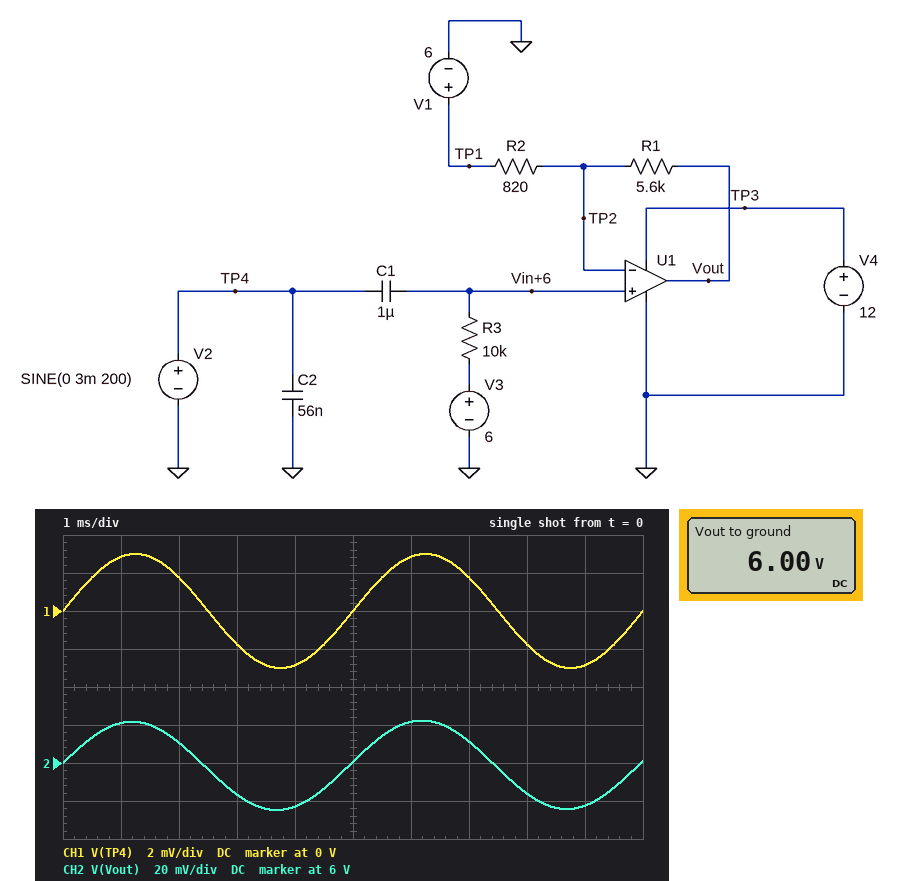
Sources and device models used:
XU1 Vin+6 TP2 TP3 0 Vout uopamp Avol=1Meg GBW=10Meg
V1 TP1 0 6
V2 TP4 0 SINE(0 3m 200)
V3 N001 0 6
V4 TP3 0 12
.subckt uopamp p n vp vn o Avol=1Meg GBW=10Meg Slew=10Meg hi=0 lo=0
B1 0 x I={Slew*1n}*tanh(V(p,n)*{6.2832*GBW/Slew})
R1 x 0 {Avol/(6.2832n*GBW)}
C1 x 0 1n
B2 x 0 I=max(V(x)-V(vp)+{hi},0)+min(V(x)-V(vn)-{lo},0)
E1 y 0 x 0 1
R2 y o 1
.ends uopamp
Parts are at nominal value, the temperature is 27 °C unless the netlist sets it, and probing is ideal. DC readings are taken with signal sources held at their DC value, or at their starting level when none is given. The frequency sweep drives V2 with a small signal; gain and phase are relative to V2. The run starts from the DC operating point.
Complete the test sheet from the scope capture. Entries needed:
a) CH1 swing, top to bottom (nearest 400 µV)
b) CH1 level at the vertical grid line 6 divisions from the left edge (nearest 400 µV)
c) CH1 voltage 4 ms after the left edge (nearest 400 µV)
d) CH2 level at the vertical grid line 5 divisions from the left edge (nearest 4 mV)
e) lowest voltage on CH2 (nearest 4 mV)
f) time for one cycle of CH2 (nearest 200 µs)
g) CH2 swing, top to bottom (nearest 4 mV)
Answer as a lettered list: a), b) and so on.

a) 6.0 mV
b) 2.8 mV
c) -2.8 mV
d) 6.000 V
e) 5.976 V
f) 5.0 ms
g) 48 mV
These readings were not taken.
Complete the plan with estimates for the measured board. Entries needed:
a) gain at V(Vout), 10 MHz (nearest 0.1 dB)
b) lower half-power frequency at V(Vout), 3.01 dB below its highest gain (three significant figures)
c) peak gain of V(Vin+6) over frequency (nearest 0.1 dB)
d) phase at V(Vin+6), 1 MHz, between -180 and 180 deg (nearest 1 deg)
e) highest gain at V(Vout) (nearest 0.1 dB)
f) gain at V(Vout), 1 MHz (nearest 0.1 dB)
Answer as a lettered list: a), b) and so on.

a) -0.1 dB
b) 15.9 Hz
c) 0 dB
d) 0 deg
e) 17.9 dB
f) 15.8 dB
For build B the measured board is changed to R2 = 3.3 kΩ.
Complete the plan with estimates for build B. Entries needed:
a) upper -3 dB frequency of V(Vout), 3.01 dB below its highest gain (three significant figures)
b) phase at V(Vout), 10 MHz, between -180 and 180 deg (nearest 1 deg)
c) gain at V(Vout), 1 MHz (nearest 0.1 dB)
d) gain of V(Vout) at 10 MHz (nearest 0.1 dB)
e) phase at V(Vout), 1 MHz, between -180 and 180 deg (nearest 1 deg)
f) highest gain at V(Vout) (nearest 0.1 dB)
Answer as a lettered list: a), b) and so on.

a) 3.71 MHz
b) -70 deg
c) 8.3 dB
d) -0.6 dB
e) -15 deg
f) 8.6 dB
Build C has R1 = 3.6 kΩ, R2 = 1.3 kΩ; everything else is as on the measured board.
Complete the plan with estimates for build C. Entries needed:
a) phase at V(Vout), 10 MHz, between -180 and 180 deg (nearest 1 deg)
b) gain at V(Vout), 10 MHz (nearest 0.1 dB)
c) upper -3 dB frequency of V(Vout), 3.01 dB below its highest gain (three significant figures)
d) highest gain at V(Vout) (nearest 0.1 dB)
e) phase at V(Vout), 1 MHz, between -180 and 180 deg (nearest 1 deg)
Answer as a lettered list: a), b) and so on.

a) -75 deg
b) -0.3 dB
c) 2.65 MHz
d) 11.5 dB
e) -21 deg
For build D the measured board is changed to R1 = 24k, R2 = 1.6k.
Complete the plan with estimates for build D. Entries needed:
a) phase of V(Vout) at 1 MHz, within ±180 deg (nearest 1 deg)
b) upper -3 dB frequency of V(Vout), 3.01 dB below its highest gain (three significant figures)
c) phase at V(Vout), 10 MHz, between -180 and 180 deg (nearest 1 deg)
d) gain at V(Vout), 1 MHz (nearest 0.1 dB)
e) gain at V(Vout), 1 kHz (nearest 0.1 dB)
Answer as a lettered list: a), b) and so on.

a) -58 deg
b) 625 kHz
c) -86 deg
d) 18.6 dB
e) 24.1 dB
